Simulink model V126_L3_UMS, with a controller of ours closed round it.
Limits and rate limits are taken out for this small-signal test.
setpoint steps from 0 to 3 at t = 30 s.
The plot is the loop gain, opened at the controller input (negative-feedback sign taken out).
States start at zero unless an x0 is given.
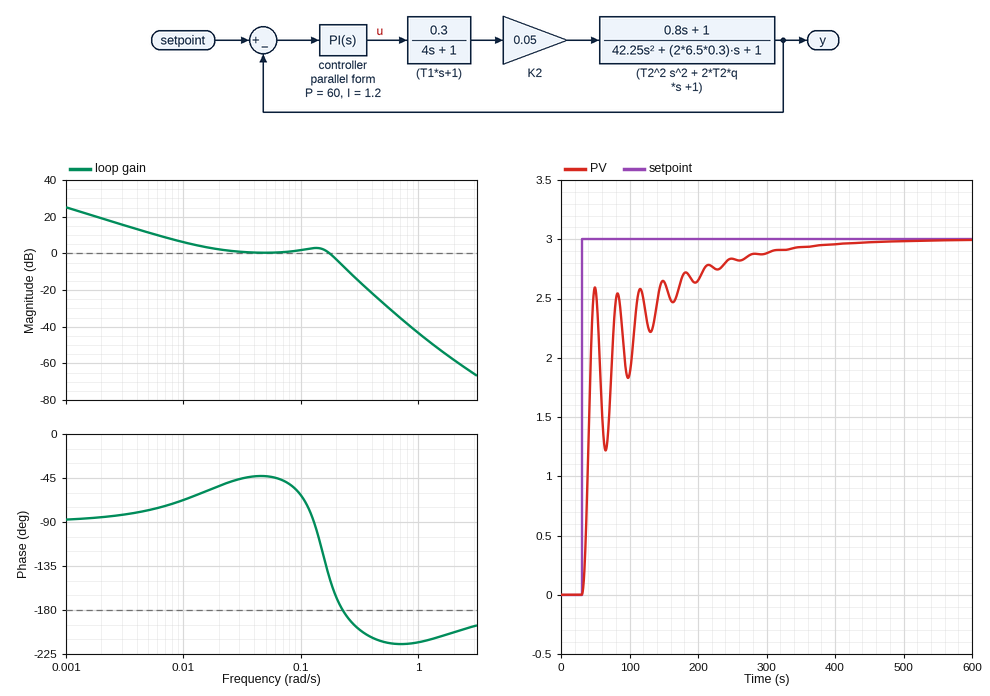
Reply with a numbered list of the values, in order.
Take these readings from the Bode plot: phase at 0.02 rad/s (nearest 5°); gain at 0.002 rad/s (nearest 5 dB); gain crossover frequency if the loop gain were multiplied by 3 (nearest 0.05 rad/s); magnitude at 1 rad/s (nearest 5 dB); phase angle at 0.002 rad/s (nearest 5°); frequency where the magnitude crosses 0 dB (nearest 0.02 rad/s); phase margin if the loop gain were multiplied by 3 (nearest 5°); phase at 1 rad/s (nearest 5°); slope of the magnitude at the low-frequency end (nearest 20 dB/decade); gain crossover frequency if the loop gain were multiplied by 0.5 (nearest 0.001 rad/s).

1. -55°
2. 20 dB
3. 0.25 rad/s
4. -45 dB
5. -85°
6. 0.18 rad/s
7. -10°
8. -215°
9. -20 dB/decade
10. 0.010 rad/s
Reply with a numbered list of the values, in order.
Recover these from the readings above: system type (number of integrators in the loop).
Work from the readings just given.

1. 1
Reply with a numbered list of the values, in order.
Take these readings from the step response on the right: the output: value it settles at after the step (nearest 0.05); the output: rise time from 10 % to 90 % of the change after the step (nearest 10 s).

1. 3.00
2. 140 s
